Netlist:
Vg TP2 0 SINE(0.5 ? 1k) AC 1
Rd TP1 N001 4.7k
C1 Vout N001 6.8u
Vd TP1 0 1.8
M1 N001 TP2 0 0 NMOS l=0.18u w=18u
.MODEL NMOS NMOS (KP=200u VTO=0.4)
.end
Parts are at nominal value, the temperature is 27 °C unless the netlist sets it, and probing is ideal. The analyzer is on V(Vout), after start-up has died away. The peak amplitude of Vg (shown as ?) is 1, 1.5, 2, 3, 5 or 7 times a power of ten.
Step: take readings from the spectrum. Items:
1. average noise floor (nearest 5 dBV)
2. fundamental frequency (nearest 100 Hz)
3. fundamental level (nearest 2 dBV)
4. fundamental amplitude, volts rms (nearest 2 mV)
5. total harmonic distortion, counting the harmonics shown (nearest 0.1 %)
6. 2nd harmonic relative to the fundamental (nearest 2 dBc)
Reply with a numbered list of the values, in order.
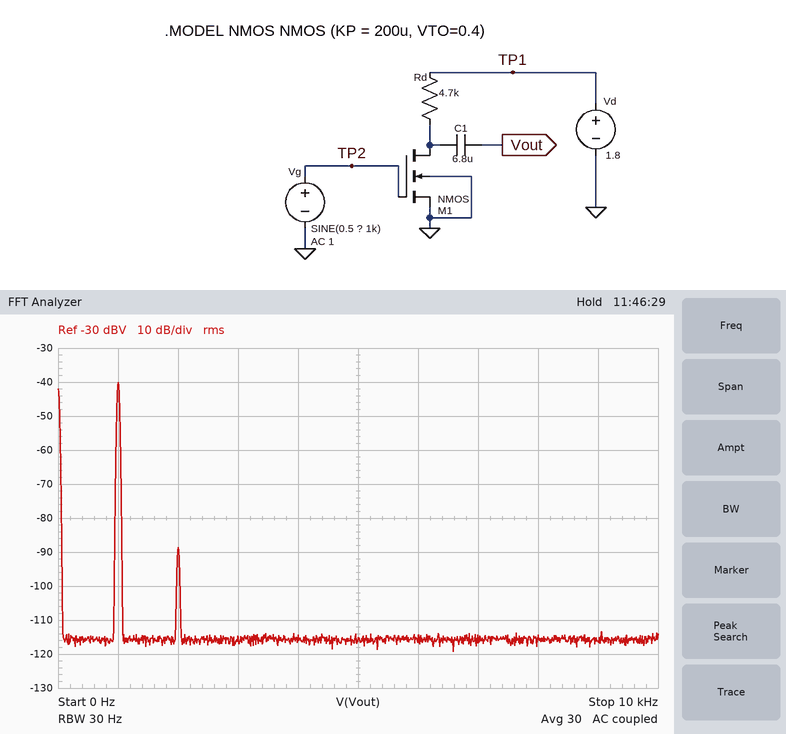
1. -115 dBV
2. 1.0 kHz
3. -40 dBV
4. 10 mV
5. 0.4 %
6. -48 dBc
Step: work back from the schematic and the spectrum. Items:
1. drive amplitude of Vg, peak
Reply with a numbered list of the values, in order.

1. 1.5 mV
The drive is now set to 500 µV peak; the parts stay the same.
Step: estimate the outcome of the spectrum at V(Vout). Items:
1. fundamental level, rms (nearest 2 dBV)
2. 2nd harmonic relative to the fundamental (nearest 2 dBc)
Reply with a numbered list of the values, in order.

1. -50 dBV
2. -58 dBc
